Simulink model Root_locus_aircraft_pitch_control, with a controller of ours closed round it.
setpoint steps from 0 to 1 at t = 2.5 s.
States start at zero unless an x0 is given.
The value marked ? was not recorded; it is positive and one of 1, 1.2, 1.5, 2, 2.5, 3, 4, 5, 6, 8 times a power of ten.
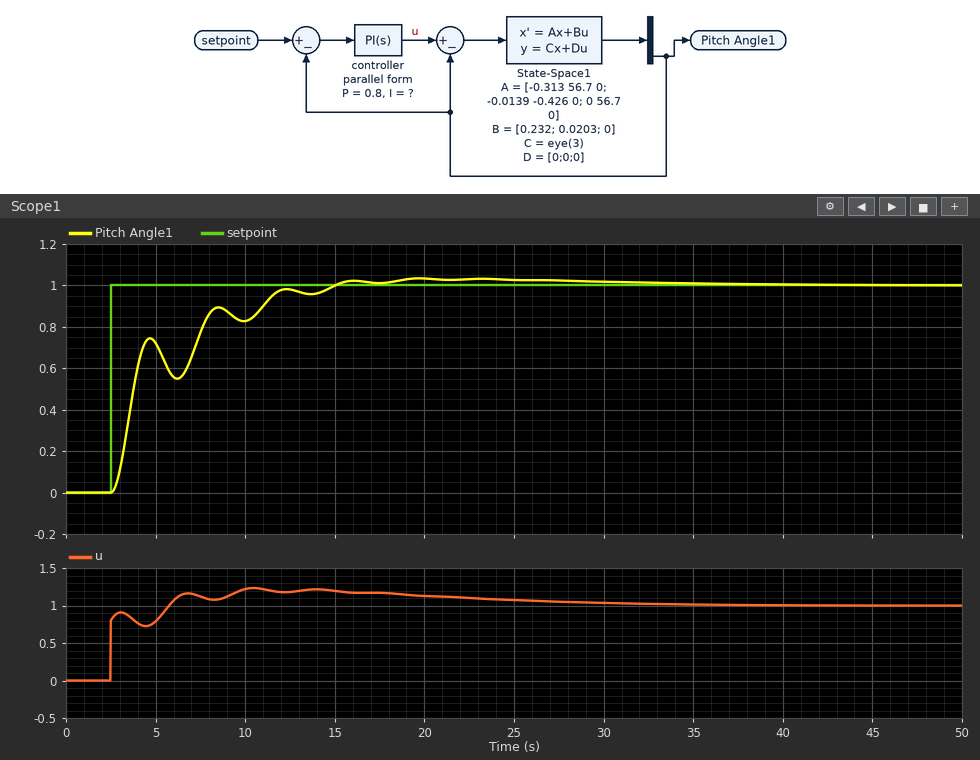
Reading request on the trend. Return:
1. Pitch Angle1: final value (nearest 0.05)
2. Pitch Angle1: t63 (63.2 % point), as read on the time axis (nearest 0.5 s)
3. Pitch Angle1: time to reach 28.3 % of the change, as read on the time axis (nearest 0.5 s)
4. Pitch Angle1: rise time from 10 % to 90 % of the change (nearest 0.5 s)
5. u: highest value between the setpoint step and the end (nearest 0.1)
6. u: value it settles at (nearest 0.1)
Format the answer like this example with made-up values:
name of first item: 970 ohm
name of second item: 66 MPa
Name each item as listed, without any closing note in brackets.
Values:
Pitch Angle1: final value: 1.00
Pitch Angle1: t63 (63.2 % point), as read on the time axis: 4.0 s
Pitch Angle1: time to reach 28.3 % of the change, as read on the time axis: 3.5 s
Pitch Angle1: rise time from 10 % to 90 % of the change: 8.0 s
u: highest value between the setpoint step and the end: 1.2
u: value it settles at: 1.0
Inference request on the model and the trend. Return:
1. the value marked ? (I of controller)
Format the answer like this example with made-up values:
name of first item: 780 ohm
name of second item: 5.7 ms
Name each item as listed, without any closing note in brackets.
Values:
the value marked ?: 0.4
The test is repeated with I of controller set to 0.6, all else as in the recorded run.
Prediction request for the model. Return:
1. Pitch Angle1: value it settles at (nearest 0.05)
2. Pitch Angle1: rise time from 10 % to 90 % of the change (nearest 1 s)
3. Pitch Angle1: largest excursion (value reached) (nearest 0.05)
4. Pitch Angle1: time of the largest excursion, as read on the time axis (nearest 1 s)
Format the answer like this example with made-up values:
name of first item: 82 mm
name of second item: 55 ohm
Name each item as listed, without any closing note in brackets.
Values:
Pitch Angle1: value it settles at: 1.00
Pitch Angle1: rise time from 10 % to 90 % of the change: 5 s
Pitch Angle1: largest excursion (value reached): 1.05
Pitch Angle1: time of the largest excursion, as read on the time axis: 12 s
